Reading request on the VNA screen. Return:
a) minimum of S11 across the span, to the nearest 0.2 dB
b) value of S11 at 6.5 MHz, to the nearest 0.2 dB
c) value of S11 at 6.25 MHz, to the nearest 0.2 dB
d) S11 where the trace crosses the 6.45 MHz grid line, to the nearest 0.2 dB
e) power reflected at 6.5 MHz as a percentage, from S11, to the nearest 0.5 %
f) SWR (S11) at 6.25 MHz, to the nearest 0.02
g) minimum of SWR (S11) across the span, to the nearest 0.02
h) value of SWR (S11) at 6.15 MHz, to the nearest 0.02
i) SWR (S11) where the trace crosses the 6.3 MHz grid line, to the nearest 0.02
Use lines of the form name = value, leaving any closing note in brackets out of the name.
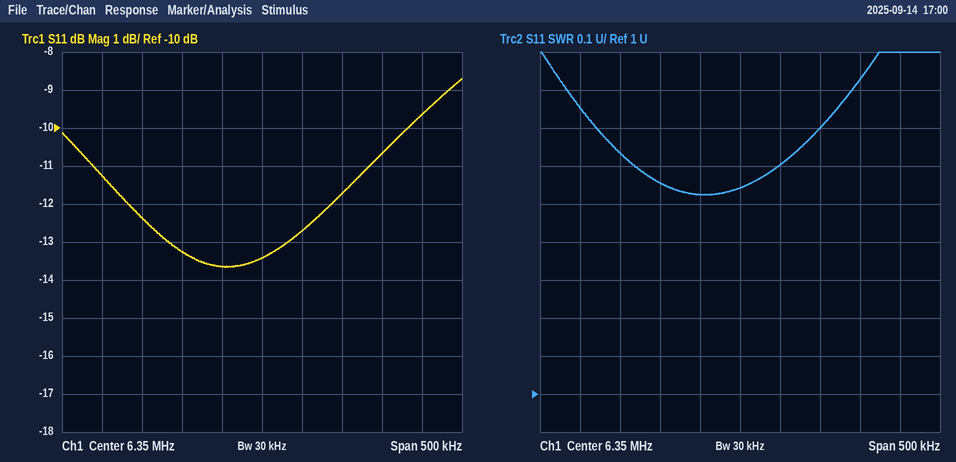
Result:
minimum of S11 across the span, to the nearest 0.2 dB = -13.6 dB
value of S11 at 6.5 MHz, to the nearest 0.2 dB = -10.6 dB
value of S11 at 6.25 MHz, to the nearest 0.2 dB = -13.2 dB
S11 where the trace crosses the 6.45 MHz grid line, to the nearest 0.2 dB = -11.8 dB
power reflected at 6.5 MHz as a percentage, from S11, to the nearest 0.5 % = 8.5 %
SWR (S11) at 6.25 MHz, to the nearest 0.02 = 1.56
minimum of SWR (S11) across the span, to the nearest 0.02 = 1.52
value of SWR (S11) at 6.15 MHz, to the nearest 0.02 = 1.76
SWR (S11) where the trace crosses the 6.3 MHz grid line, to the nearest 0.02 = 1.52
